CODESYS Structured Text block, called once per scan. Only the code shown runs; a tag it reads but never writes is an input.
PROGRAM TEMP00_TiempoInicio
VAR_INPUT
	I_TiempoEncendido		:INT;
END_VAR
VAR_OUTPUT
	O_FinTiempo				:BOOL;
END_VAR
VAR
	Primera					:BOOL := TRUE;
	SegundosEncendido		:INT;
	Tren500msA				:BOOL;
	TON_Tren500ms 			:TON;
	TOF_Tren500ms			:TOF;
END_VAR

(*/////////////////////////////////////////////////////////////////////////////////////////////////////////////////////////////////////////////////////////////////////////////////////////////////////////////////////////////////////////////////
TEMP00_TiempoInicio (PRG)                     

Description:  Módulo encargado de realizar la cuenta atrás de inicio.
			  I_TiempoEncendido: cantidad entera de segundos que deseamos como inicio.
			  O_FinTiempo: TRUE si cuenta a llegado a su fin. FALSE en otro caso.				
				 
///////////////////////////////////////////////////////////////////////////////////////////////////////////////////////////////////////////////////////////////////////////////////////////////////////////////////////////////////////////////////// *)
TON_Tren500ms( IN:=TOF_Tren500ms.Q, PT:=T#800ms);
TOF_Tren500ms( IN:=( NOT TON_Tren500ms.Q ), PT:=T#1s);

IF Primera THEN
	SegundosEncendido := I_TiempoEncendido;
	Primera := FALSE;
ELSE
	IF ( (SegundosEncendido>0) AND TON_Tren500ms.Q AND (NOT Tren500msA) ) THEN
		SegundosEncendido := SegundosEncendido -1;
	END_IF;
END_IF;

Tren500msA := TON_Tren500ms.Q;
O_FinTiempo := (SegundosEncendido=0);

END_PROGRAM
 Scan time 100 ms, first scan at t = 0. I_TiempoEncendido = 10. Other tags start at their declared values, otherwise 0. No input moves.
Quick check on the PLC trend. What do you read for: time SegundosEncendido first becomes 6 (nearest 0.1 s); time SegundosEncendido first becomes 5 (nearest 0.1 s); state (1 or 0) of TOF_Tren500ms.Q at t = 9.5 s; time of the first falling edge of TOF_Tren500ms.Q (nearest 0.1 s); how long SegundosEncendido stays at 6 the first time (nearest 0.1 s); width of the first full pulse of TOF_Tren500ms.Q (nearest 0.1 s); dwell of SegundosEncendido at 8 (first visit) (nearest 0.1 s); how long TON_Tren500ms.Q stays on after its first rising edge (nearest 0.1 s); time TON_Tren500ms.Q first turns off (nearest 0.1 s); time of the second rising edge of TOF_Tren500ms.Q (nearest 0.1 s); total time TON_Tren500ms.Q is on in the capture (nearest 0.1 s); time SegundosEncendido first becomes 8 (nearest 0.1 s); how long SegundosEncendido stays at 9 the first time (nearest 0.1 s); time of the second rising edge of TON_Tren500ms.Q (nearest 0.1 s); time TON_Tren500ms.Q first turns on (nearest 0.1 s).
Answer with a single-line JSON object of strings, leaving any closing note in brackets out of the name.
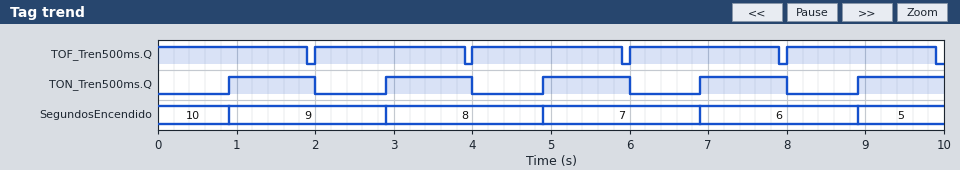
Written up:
{"time SegundosEncendido first becomes 6": "6.9 s", "time SegundosEncendido first becomes 5": "8.9 s", "state (1 or 0) of TOF_Tren500ms.Q at t = 9.5 s": "1", "time of the first falling edge of TOF_Tren500ms.Q": "1.9 s", "how long SegundosEncendido stays at 6 the first time": "2.0 s", "width of the first full pulse of TOF_Tren500ms.Q": "1.9 s", "dwell of SegundosEncendido at 8 (first visit)": "2.0 s", "how long TON_Tren500ms.Q stays on after its first rising edge": "1.1 s", "time TON_Tren500ms.Q first turns off": "2.0 s", "time of the second rising edge of TOF_Tren500ms.Q": "4.0 s", "total time TON_Tren500ms.Q is on in the capture": "5.5 s", "time SegundosEncendido first becomes 8": "2.9 s", "how long SegundosEncendido stays at 9 the first time": "2.0 s", "time of the second rising edge of TON_Tren500ms.Q": "2.9 s", "time TON_Tren500ms.Q first turns on": "0.9 s"}
